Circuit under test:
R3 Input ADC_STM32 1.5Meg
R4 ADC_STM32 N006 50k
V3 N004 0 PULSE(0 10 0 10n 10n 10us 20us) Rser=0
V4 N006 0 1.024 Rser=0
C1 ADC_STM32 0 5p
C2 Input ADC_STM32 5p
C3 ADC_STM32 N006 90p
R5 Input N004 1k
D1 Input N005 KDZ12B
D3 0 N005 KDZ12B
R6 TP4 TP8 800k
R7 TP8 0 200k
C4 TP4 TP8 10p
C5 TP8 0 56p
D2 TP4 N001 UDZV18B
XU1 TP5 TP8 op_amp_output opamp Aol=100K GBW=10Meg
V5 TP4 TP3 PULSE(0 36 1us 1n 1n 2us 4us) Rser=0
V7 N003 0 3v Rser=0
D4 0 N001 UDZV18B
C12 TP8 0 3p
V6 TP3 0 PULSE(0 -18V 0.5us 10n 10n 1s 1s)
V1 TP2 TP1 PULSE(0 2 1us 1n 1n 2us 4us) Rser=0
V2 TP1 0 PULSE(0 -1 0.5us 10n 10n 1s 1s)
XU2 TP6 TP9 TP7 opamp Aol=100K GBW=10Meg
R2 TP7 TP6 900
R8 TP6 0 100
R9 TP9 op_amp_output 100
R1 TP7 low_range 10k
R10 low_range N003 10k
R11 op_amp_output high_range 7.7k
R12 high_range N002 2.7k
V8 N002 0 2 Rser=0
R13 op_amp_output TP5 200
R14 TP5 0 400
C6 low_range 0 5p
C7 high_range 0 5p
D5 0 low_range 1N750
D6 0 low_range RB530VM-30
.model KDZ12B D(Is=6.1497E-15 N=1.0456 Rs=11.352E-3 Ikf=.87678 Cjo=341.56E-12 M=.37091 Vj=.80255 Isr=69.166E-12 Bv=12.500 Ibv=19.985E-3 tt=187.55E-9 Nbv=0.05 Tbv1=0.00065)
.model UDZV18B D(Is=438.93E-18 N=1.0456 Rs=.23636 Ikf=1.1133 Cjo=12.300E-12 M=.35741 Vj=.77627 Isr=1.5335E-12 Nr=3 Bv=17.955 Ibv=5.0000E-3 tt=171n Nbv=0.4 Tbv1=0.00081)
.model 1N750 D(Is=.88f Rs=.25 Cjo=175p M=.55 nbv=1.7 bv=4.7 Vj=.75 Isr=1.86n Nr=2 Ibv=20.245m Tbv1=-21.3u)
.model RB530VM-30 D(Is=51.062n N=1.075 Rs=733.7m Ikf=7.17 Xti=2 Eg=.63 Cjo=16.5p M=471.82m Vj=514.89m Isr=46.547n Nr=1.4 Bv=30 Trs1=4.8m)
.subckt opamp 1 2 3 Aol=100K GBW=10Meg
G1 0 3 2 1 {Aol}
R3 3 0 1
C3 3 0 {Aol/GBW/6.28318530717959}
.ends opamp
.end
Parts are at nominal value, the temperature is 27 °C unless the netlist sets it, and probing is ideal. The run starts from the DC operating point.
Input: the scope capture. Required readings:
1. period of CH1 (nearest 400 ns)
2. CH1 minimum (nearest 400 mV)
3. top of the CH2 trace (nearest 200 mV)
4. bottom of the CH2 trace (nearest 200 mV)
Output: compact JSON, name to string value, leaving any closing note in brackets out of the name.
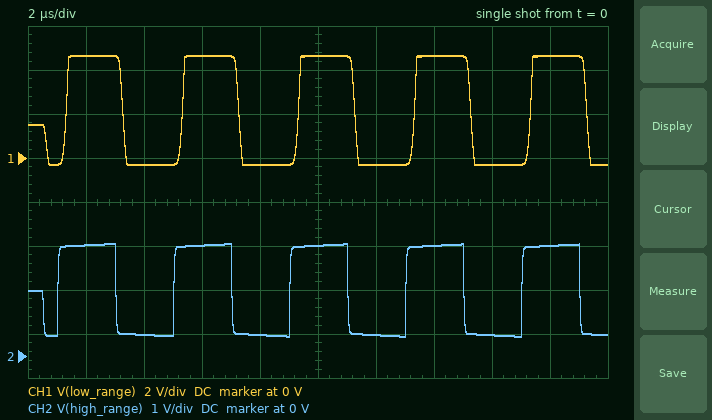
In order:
{"period of CH1": "4.0 µs", "CH1 minimum": "-400 mV", "top of the CH2 trace": "2.6 V", "bottom of the CH2 trace": "400 mV"}
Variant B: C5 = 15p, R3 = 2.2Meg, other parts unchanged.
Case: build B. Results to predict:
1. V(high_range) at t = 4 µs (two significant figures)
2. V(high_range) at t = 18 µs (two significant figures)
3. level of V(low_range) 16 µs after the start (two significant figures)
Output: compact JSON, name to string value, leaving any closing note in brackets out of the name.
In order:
{"V(high_range) at t = 4 µs": "-1.1 V", "V(high_range) at t = 18 µs": "4.0 V", "level of V(low_range) 16 µs after the start": "-340 mV"}
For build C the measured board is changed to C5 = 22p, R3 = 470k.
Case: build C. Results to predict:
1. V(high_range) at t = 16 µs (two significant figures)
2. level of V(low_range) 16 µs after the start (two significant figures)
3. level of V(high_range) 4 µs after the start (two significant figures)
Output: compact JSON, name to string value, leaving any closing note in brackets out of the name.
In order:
{"V(high_range) at t = 16 µs": "-520 mV", "level of V(low_range) 16 µs after the start": "-340 mV", "level of V(high_range) 4 µs after the start": "-550 mV"}
